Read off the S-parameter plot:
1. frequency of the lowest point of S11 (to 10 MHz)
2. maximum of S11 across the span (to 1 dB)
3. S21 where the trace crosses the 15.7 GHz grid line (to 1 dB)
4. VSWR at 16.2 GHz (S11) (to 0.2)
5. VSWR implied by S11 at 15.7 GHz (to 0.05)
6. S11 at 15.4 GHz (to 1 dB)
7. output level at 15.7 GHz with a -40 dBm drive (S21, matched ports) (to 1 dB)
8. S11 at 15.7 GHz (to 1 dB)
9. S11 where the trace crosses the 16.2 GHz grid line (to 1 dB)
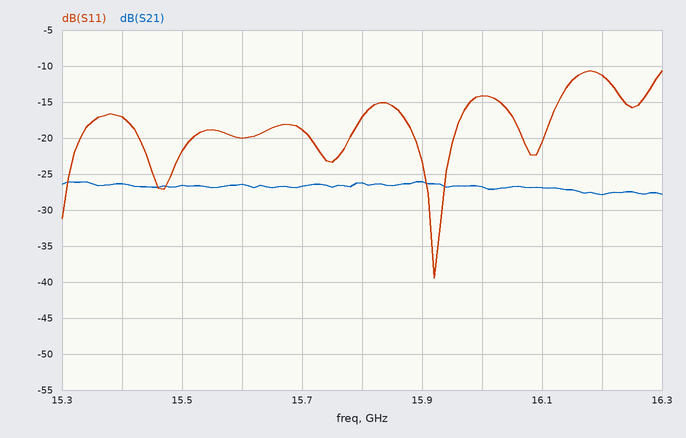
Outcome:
15.92 GHz
-11 dB
-27 dB
1.8
1.25
-17 dB
-67 dBm
-19 dB
-11 dB
